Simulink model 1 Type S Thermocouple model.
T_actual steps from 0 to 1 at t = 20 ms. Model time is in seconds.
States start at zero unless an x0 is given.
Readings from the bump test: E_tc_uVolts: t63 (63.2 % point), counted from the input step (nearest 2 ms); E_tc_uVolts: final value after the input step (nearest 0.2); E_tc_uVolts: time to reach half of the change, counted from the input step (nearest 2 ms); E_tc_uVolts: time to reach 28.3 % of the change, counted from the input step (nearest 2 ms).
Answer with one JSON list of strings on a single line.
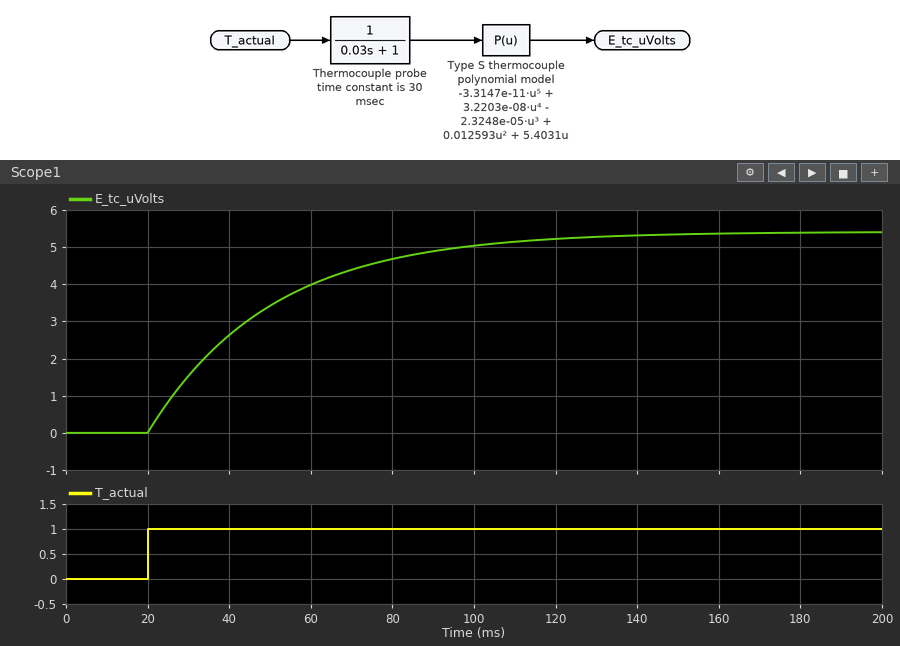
["30 ms", "5.4", "20 ms", "10 ms"]
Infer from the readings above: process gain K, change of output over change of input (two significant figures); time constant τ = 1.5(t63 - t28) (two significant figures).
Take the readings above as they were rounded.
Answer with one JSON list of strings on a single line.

["5.4", "30 ms"]
